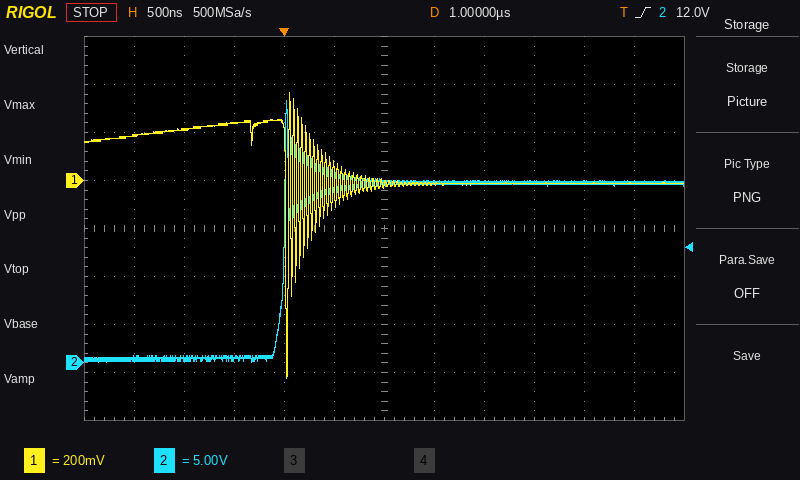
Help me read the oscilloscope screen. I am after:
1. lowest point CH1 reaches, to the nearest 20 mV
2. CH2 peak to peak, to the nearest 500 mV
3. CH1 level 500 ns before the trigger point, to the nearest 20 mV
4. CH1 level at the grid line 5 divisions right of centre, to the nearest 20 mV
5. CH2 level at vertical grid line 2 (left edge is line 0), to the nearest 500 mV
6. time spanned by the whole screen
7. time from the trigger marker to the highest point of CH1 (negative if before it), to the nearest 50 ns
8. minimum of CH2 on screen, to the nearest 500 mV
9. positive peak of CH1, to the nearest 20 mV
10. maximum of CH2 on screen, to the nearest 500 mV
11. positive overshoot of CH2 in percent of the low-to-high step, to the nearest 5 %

-820 mV
27.5 V
240 mV
-20 mV
500 mV
6 µs
+50 ns
0.0 V
360 mV
27.5 V
45 %
